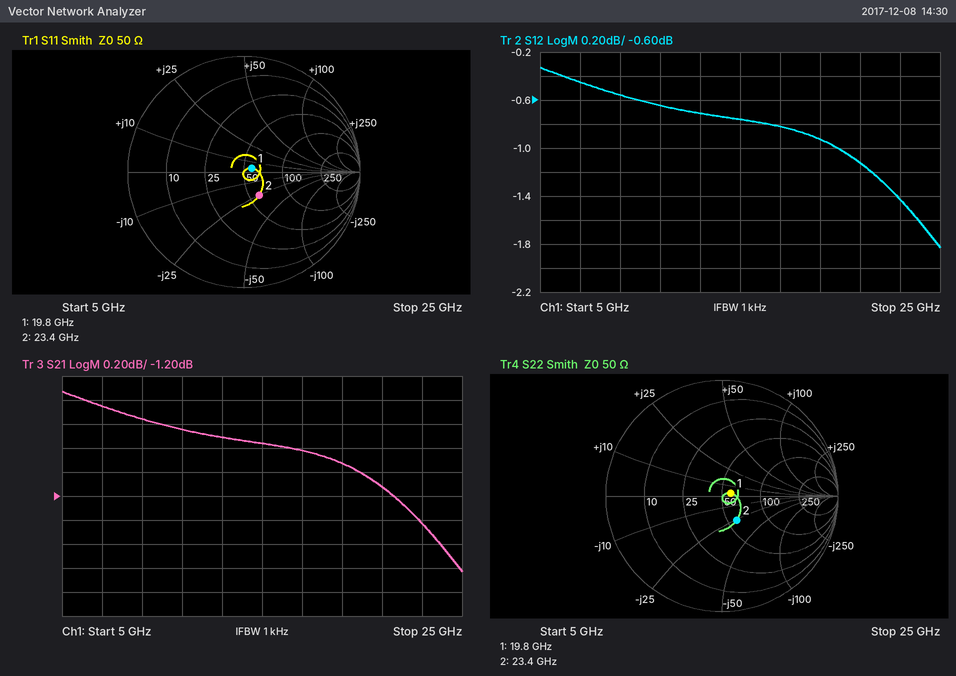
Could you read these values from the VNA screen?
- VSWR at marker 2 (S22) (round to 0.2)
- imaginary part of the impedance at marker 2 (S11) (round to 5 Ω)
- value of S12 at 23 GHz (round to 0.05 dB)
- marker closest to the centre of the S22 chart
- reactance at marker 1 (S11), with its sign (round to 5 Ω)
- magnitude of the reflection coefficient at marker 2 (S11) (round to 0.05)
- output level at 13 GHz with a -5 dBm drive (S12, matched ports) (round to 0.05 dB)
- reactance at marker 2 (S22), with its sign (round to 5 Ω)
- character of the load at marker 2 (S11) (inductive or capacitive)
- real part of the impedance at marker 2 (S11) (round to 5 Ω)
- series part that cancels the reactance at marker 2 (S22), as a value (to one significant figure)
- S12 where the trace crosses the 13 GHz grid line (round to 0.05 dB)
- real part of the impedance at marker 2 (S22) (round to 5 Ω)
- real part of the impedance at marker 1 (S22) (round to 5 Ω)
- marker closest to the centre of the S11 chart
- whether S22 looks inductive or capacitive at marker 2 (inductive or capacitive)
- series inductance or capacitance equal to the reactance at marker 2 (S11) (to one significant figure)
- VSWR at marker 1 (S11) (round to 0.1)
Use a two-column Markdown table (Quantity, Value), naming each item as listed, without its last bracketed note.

| Quantity | Value |
|---|---|
| VSWR at marker 2 (S22) | 1.6 |
| imaginary part of the impedance at marker 2 (S11) | -25 Ω |
| value of S12 at 23 GHz | -1.45 dB |
| marker closest to the centre of the S22 chart | marker 1 |
| reactance at marker 1 (S11), with its sign | +5 Ω |
| magnitude of the reflection coefficient at marker 2 (S11) | 0.25 |
| output level at 13 GHz with a -5 dBm drive (S12, matched ports) | -5.70 dBm |
| reactance at marker 2 (S22), with its sign | -25 Ω |
| character of the load at marker 2 (S11) | capacitive |
| real part of the impedance at marker 2 (S11) | 60 Ω |
| series part that cancels the reactance at marker 2 (S22), as a value | 200 pH |
| S12 where the trace crosses the 13 GHz grid line | -0.70 dB |
| real part of the impedance at marker 2 (S22) | 60 Ω |
| real part of the impedance at marker 1 (S22) | 60 Ω |
| marker closest to the centre of the S11 chart | marker 1 |
| whether S22 looks inductive or capacitive at marker 2 | capacitive |
| series inductance or capacitance equal to the reactance at marker 2 (S11) | 300 fF |
| VSWR at marker 1 (S11) | 1.2 |
